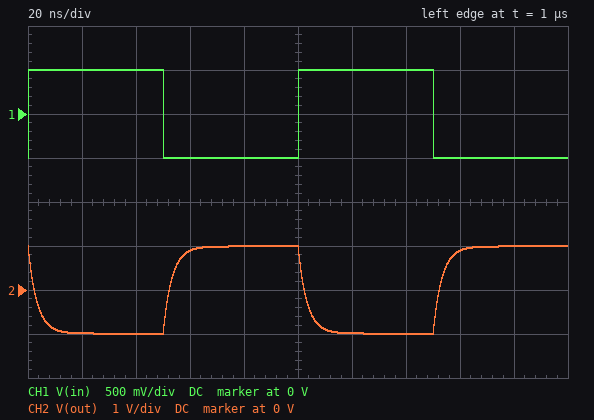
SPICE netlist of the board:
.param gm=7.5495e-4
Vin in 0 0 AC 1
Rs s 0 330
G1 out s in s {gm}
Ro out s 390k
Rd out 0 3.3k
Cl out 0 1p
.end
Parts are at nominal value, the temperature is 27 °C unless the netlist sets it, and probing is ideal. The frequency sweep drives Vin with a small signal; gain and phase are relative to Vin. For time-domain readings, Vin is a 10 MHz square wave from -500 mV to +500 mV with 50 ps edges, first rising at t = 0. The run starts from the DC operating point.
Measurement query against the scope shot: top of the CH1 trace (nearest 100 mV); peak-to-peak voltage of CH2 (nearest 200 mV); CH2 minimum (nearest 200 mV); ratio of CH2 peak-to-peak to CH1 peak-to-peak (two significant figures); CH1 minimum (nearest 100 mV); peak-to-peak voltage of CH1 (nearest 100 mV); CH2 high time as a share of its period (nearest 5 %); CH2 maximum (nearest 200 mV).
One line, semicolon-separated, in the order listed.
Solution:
500 mV; 2.0 V; -1.0 V; 2.0; -500 mV; 1.0 V; 50 %; 1.0 V
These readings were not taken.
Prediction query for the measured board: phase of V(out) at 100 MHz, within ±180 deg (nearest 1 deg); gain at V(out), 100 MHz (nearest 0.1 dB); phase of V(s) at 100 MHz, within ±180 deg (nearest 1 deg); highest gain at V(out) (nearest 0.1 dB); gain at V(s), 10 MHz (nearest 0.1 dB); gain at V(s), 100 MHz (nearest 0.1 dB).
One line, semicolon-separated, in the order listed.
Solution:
116 deg; -1.3 dB; 0 deg; 5.9 dB; -14.1 dB; -14.0 dB
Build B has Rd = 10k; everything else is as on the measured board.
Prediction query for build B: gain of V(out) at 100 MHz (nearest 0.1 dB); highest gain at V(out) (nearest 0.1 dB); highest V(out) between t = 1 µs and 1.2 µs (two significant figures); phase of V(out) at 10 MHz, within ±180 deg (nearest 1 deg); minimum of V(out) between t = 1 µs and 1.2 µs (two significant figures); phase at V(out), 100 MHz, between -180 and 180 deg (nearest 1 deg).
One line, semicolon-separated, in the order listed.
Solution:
-0.5 dB; 15.4 dB; 2.9 V; 148 deg; -2.9 V; 99 deg
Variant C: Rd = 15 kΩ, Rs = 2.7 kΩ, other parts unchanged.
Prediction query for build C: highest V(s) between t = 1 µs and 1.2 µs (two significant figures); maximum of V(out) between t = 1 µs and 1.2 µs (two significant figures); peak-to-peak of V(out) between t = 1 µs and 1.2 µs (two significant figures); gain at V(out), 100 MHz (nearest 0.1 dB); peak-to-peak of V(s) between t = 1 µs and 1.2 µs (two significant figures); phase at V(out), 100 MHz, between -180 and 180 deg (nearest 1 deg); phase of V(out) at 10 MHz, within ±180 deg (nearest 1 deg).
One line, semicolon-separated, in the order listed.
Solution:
340 mV; 1.7 V; 3.4 V; -8.1 dB; 680 mV; 96 deg; 137 deg
